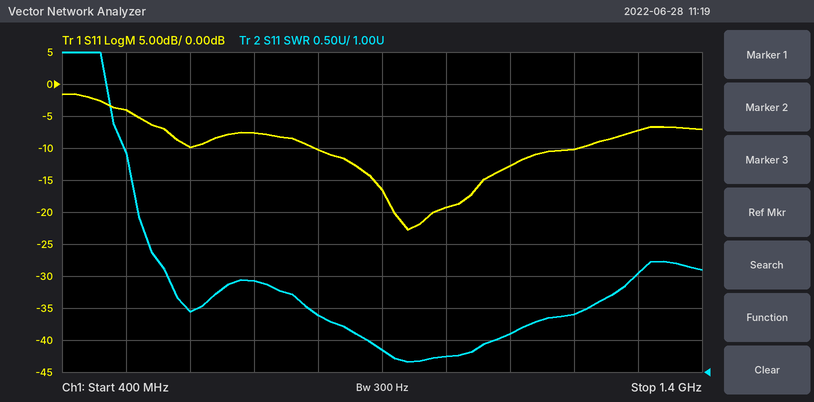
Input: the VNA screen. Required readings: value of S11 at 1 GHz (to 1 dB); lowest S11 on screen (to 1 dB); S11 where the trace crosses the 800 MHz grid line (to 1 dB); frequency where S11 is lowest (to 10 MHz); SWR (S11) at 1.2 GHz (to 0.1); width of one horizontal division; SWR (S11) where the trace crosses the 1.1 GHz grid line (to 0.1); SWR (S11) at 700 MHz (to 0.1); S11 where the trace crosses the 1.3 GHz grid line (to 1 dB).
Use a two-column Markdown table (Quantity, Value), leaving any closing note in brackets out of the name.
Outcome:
| Quantity | Value |
|---|---|
| value of S11 at 1 GHz | -19 dB |
| lowest S11 on screen | -23 dB |
| S11 where the trace crosses the 800 MHz grid line | -10 dB |
| frequency where S11 is lowest | 940 MHz |
| SWR (S11) at 1.2 GHz | 1.9 |
| width of one horizontal division | 100 MHz |
| SWR (S11) where the trace crosses the 1.1 GHz grid line | 1.6 |
| SWR (S11) at 700 MHz | 2.4 |
| S11 where the trace crosses the 1.3 GHz grid line | -7 dB |
